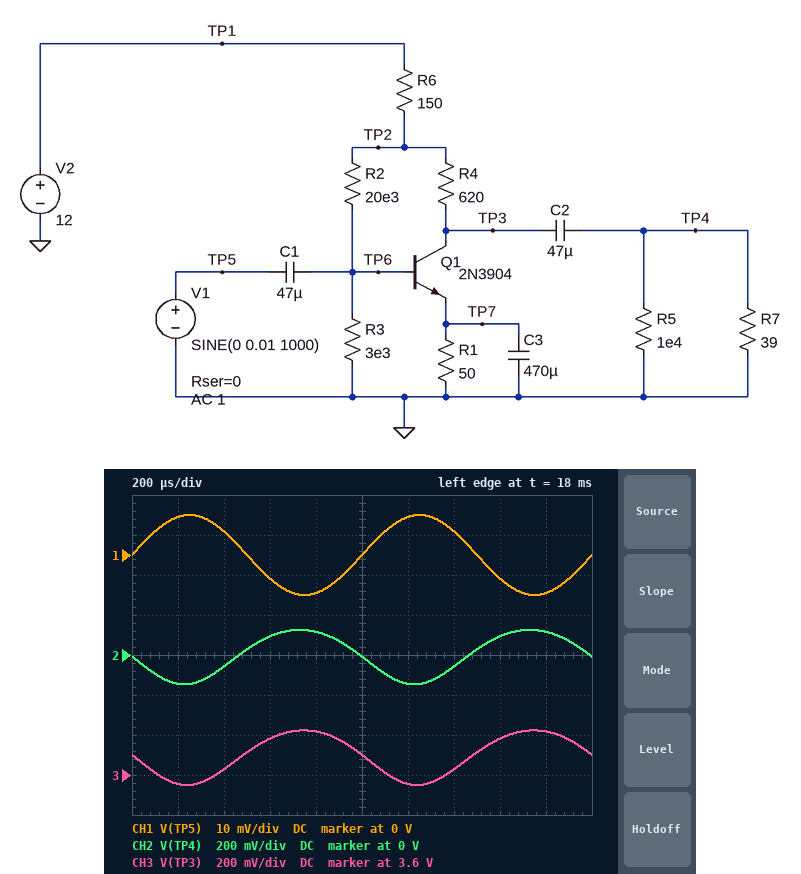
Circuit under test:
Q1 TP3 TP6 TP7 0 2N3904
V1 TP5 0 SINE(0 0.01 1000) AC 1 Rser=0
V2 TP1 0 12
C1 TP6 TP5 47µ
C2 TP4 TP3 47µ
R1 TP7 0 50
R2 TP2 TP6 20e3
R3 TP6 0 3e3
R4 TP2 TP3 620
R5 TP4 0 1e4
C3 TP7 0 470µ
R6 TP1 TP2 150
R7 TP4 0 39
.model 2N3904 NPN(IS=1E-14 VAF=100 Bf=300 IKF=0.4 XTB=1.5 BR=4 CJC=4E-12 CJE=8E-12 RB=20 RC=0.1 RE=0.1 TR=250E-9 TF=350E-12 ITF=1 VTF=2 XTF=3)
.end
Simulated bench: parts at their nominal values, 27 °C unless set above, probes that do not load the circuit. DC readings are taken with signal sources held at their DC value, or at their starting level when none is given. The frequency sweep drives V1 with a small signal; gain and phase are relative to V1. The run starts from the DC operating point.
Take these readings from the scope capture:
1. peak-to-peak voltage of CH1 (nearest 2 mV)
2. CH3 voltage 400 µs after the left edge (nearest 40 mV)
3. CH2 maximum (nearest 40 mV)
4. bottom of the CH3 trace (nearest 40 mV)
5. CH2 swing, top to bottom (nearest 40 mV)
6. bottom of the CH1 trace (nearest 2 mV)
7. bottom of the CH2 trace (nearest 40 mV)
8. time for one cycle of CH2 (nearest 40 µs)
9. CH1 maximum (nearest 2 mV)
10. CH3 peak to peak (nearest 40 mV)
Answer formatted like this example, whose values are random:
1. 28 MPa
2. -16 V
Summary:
1. 20 mV
2. 3.64 V
3. 120 mV
4. 3.56 V
5. 280 mV
6. -10 mV
7. -160 mV
8. 1.00 ms
9. 10 mV
10. 280 mV
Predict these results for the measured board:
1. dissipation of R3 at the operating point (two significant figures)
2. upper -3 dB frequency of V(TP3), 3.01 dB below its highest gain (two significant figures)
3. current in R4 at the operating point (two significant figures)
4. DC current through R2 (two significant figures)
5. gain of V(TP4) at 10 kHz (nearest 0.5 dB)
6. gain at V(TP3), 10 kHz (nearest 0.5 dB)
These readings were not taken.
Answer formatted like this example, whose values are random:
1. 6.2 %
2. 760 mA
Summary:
1. 520 µW
2. 44 MHz
3. 11 mA
4. 450 µA
5. 23.0 dB
6. 23.0 dB
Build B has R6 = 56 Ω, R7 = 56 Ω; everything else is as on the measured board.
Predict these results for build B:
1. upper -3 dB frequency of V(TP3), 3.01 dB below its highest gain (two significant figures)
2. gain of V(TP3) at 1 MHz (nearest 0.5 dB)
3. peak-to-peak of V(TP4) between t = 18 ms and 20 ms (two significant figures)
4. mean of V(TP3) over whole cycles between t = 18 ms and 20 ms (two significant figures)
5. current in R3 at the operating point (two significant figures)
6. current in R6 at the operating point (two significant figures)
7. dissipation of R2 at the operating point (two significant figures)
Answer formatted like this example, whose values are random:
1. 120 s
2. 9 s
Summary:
1. 35 MHz
2. 27.0 dB
3. 440 mV
4. 3.4 V
5. 450 µA
6. 13 mA
7. 4.9 mW
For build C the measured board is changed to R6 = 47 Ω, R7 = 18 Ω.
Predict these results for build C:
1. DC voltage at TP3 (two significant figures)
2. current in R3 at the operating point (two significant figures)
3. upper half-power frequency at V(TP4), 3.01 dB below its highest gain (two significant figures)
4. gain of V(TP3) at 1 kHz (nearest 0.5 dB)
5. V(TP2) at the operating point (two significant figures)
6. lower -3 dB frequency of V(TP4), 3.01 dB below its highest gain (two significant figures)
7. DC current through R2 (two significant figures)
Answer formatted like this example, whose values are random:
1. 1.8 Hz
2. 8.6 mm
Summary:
1. 3.4 V
2. 460 µA
3. 41 MHz
4. 18.0 dB
5. 11 V
6. 160 Hz
7. 500 µA
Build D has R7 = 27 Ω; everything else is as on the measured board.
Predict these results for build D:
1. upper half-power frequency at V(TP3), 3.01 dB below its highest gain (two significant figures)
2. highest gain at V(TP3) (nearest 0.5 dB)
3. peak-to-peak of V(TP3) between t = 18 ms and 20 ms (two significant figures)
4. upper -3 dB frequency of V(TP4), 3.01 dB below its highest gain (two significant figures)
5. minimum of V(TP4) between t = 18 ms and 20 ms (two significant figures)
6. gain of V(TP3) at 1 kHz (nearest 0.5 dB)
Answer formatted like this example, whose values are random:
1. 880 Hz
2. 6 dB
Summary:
1. 35 MHz
2. 21.0 dB
3. 190 mV
4. 46 MHz
5. -100 mV
6. 20.0 dB
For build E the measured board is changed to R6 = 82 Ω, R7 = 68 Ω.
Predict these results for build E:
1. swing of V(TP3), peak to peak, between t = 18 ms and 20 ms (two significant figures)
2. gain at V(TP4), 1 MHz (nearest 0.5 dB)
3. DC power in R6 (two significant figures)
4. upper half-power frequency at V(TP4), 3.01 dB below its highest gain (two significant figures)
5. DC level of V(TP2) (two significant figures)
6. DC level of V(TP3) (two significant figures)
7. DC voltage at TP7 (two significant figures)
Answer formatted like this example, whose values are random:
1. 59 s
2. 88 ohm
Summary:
1. 500 mV
2. 28.0 dB
3. 13 mW
4. 35 MHz
5. 11 V
6. 3.5 V
7. 600 mV
